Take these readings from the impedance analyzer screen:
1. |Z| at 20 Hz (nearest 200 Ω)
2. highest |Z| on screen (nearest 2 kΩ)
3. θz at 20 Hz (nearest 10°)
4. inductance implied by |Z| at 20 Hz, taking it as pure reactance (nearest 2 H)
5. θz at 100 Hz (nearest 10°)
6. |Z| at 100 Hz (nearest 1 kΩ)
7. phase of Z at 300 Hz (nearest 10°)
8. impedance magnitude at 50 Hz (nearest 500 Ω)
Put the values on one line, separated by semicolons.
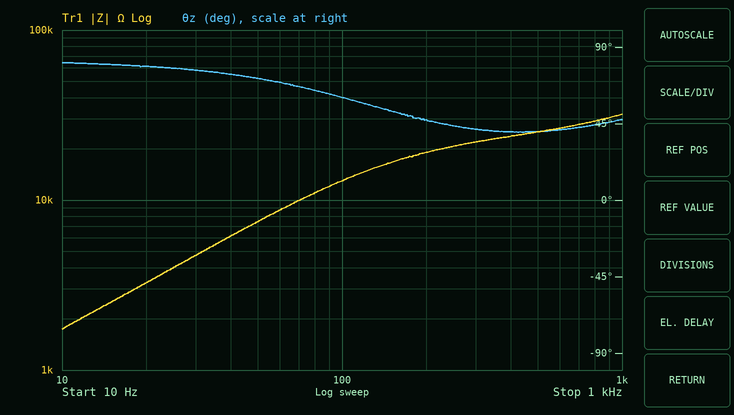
3.2 kΩ; 32 kΩ; 80°; 26 H; 60°; 13 kΩ; 40°; 7.5 kΩ
